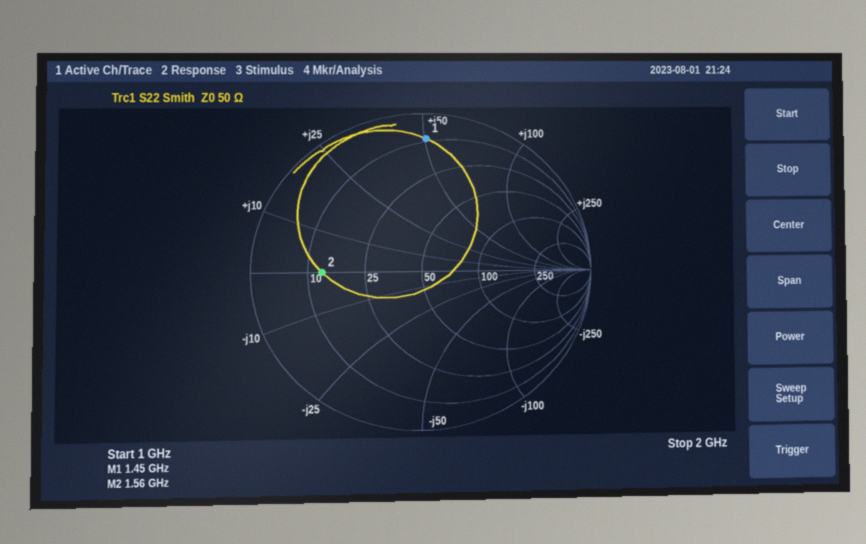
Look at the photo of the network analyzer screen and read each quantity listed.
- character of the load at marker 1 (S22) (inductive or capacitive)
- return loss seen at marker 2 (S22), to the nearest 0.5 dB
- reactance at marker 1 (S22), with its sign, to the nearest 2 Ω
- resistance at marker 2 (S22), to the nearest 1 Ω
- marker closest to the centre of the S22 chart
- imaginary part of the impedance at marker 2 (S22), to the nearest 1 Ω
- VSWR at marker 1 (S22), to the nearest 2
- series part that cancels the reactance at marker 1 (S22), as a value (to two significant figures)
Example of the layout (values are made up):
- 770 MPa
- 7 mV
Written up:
- inductive
- 4.5 dB
- +50 Ω
- 13 Ω
- marker 2
- 0 Ω
- 12
- 2.2 pF
